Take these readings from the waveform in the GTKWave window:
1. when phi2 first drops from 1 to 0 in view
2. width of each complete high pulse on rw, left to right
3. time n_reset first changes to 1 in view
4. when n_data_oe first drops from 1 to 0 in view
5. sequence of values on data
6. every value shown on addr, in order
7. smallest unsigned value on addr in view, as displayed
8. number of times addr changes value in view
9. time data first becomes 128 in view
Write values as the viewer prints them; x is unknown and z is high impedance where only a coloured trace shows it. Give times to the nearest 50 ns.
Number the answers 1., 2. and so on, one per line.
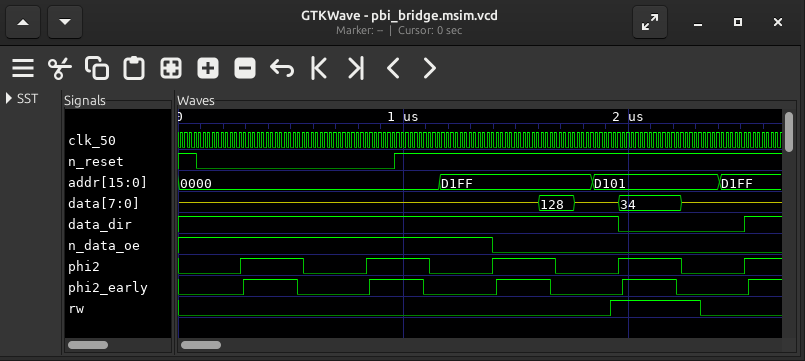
1. 550 ns
2. 400 ns
3. 950 ns
4. 1400 ns
5. z, 128, z, 34, z
6. 0000, D1FF, D101, D1FF
7. 0000
8. 3
9. 1600 ns
